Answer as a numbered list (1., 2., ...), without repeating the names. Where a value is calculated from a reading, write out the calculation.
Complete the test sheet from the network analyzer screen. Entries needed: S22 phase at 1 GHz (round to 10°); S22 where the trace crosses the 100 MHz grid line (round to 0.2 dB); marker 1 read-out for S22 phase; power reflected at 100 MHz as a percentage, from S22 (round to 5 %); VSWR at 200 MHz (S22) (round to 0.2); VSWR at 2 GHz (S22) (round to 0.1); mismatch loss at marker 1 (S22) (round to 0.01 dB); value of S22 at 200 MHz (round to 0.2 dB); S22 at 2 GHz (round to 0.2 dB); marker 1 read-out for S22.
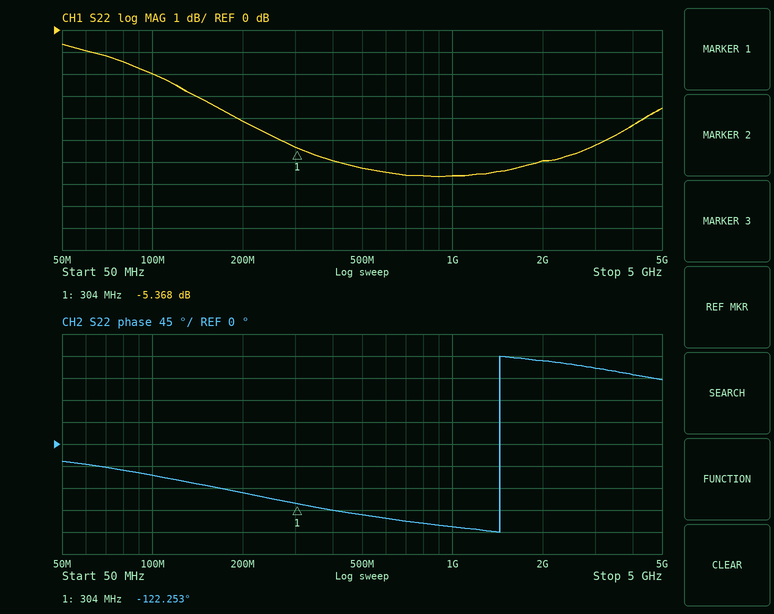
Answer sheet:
1. -170°
2. -2.0 dB
3. -122.253°
4. 10^(-2/10) ≈ 63.1 %, so 65 % to the nearest 5 %
5. |Γ| = 10^(-4.2/20) = 0.6166; VSWR = (1 + 0.6166)/(1 − 0.6166) ≈ 4.2
6. |Γ| = 10^(-6/20) = 0.5012; VSWR = (1 + 0.5012)/(1 − 0.5012) ≈ 3.0
7. −10 log10(1 − 10^(-5.368/10)) ≈ 1.49 dB
8. -4.2 dB
9. -6.0 dB
10. -5.368 dB
